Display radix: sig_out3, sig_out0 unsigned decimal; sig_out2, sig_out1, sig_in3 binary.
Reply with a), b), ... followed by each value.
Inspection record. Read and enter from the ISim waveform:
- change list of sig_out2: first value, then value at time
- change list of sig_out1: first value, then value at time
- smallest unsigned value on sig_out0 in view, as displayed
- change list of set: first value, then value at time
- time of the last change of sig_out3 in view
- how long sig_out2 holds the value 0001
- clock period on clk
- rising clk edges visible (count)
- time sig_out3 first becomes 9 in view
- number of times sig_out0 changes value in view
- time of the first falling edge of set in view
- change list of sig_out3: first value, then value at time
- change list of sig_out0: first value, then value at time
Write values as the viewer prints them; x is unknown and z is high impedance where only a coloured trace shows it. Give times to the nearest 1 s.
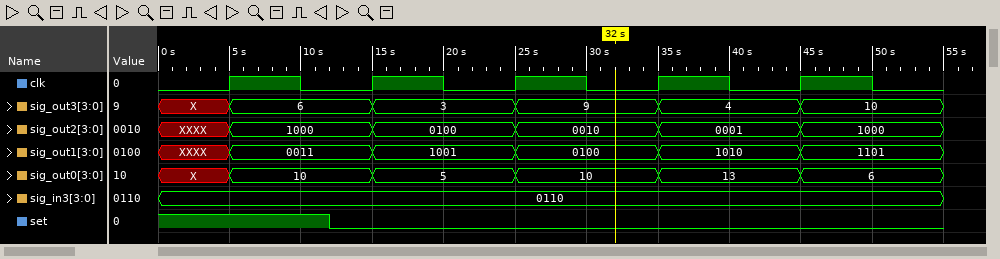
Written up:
a) XXXX, 1000 at 5 s, 0100 at 15 s, 0010 at 25 s, 0001 at 35 s, 1000 at 45 s
b) XXXX, 0011 at 5 s, 1001 at 15 s, 0100 at 25 s, 1010 at 35 s, 1101 at 45 s
c) 5
d) 1, 0 at 12 s
e) 45 s
f) 10 s
g) 10 s
h) 5
i) 25 s
j) 5
k) 12 s
l) X, 6 at 5 s, 3 at 15 s, 9 at 25 s, 4 at 35 s, 10 at 45 s
m) X, 10 at 5 s, 5 at 15 s, 10 at 25 s, 13 at 35 s, 6 at 45 s
